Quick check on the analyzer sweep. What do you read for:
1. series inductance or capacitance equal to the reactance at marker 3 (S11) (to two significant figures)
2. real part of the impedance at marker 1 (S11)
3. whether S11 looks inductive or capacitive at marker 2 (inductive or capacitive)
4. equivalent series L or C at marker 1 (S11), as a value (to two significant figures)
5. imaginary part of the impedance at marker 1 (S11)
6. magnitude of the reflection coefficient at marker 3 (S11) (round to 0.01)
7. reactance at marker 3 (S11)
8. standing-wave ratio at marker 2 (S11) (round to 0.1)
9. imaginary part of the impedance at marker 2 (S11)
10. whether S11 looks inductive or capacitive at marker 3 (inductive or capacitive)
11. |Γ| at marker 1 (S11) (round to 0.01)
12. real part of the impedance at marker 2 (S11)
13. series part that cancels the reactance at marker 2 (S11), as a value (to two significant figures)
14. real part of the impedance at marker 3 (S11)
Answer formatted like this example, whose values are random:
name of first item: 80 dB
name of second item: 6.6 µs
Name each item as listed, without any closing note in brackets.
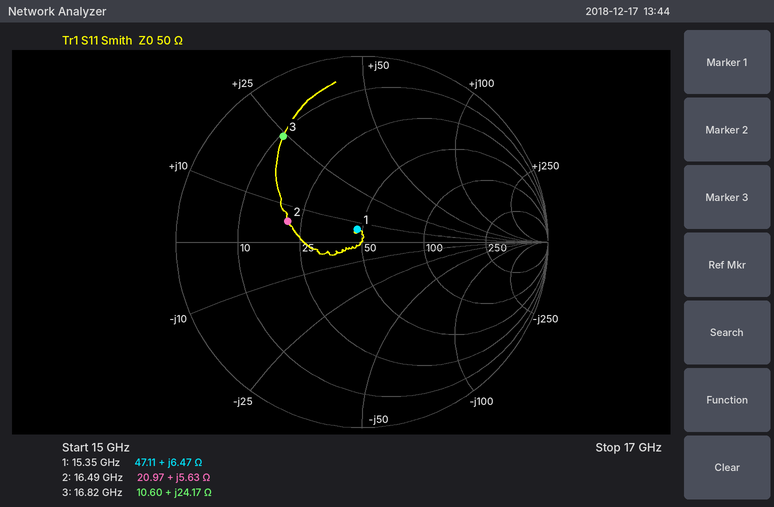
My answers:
series inductance or capacitance equal to the reactance at marker 3 (S11): 230 pH
real part of the impedance at marker 1: 47.11 Ω
whether S11 looks inductive or capacitive at marker 2: inductive
equivalent series L or C at marker 1 (S11), as a value: 67 pH
imaginary part of the impedance at marker 1: +6.47 Ω
magnitude of the reflection coefficient at marker 3 (S11): 0.71
reactance at marker 3: +24.17 Ω
standing-wave ratio at marker 2 (S11): 2.4
imaginary part of the impedance at marker 2: +5.63 Ω
whether S11 looks inductive or capacitive at marker 3: inductive
|Γ| at marker 1 (S11): 0.07
real part of the impedance at marker 2: 20.97 Ω
series part that cancels the reactance at marker 2 (S11), as a value: 1.7 pF
real part of the impedance at marker 3: 10.60 Ω
